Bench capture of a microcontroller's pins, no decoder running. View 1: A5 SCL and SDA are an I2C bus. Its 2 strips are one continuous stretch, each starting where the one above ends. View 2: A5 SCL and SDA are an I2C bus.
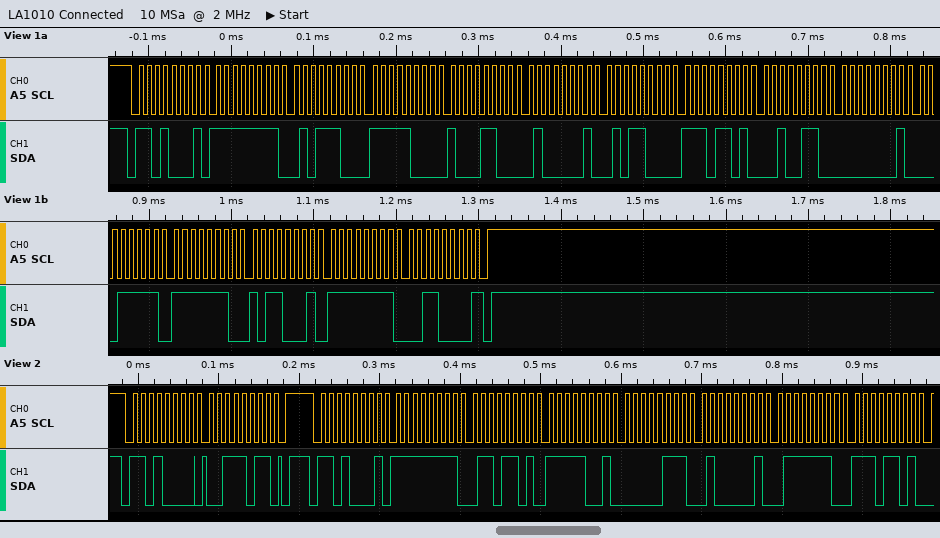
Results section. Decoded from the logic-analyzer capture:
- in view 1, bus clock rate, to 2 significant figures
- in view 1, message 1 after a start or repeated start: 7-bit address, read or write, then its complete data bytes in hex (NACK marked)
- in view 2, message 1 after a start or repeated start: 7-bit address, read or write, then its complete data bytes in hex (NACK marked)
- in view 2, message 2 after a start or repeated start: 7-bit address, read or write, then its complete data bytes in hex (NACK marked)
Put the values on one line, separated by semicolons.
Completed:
100 kHz; 0x68 read: FF 5C F8 8C 41 58 ED 26 01 1F FE B1 FF 30 NACK; 0x68 write: 3B; 0x68 read: FF 6D F9 07 41 7E ED
